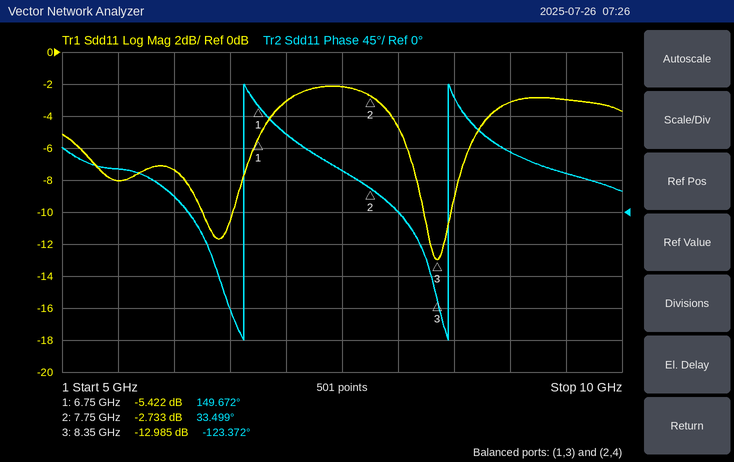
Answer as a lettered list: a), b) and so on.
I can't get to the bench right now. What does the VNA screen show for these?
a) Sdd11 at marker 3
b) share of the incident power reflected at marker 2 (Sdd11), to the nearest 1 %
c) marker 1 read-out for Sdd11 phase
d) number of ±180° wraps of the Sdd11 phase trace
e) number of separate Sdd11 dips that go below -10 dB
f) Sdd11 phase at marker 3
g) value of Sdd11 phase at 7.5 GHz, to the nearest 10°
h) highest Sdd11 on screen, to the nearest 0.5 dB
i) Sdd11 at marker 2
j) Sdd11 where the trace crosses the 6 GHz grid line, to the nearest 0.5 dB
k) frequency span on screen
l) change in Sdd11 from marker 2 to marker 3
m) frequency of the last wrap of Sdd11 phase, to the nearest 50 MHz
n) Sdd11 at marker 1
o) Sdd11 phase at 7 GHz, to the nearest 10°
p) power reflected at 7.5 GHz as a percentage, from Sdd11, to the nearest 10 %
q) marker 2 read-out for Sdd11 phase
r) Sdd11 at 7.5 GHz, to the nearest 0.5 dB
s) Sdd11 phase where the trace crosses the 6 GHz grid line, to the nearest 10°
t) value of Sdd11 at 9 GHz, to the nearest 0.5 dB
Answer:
a) -12.985 dB
b) 53 %
c) 149.672°
d) 2
e) 2
f) -123.372°
g) 60°
h) -2.0 dB
i) -2.733 dB
j) -7.5 dB
k) 5 GHz
l) -10.252 dB
m) 8.45 GHz
n) -5.422 dB
o) 110°
p) 60 %
q) 33.499°
r) -2.0 dB
s) 20°
t) -3.0 dB
